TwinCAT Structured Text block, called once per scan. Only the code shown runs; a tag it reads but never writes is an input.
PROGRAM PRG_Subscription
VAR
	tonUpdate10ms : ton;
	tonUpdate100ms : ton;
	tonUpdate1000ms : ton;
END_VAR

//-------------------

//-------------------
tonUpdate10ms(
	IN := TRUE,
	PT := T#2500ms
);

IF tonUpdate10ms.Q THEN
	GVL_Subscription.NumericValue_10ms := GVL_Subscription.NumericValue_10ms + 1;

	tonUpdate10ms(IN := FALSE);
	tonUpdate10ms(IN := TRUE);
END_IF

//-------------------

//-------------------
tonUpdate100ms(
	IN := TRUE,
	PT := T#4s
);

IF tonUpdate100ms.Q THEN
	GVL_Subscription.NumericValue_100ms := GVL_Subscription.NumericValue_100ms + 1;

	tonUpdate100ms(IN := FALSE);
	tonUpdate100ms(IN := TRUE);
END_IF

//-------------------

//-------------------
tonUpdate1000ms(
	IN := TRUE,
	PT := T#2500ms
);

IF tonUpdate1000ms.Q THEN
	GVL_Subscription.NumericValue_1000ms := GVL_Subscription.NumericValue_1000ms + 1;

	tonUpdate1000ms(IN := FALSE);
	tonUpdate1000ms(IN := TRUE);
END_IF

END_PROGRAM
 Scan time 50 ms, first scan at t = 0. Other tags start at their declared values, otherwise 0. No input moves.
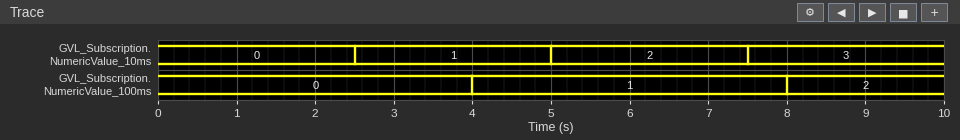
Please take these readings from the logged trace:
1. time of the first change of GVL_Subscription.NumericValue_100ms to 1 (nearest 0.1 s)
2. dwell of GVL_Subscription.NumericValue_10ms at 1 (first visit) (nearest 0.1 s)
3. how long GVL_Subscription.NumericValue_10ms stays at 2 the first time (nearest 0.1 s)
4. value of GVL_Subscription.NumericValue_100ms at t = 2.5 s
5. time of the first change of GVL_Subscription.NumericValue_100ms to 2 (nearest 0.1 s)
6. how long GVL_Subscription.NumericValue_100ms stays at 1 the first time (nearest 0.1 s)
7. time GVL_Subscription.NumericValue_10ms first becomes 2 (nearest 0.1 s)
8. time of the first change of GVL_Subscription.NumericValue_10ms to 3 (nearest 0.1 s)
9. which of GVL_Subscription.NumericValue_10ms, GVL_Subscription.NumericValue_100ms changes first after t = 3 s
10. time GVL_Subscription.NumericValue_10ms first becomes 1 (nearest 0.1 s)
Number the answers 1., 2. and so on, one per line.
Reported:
1. 4.0 s
2. 2.5 s
3. 2.5 s
4. 0
5. 8.0 s
6. 4.0 s
7. 5.0 s
8. 7.5 s
9. GVL_Subscription.NumericValue_100ms
10. 2.5 s
